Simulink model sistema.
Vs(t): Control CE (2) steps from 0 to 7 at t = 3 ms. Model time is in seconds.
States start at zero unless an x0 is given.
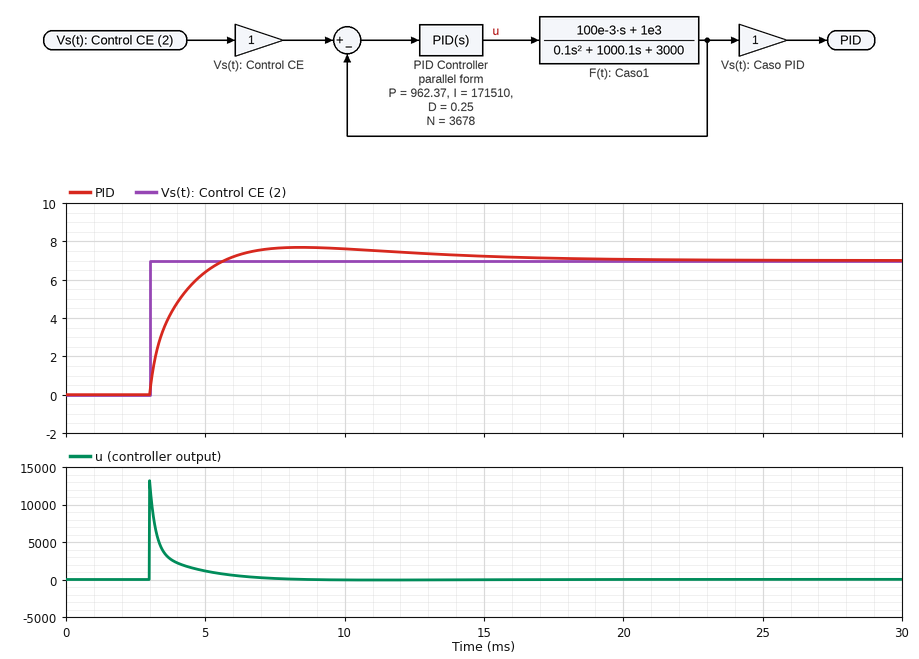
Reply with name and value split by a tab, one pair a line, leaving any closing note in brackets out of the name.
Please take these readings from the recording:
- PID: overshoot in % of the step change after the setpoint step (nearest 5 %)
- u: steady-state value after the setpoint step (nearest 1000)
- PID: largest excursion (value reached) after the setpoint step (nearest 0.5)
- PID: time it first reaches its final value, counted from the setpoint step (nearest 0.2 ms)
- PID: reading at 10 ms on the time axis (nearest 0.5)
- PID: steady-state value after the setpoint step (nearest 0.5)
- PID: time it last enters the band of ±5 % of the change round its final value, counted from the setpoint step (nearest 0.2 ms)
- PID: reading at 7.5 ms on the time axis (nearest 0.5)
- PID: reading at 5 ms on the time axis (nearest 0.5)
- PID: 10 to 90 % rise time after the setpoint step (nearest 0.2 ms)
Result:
PID: overshoot in % of the step change after the setpoint step	10 %
u: steady-state value after the setpoint step	0
PID: largest excursion (value reached) after the setpoint step	7.5
PID: time it first reaches its final value, counted from the setpoint step	2.6 ms
PID: reading at 10 ms on the time axis	7.5
PID: steady-state value after the setpoint step	7.0
PID: time it last enters the band of ±5 % of the change round its final value, counted from the setpoint step	10.0 ms
PID: reading at 7.5 ms on the time axis	7.5
PID: reading at 5 ms on the time axis	6.5
PID: 10 to 90 % rise time after the setpoint step	1.8 ms
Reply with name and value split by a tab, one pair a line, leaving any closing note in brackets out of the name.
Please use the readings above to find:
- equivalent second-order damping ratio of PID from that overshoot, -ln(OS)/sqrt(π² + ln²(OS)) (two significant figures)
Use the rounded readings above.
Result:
equivalent second-order damping ratio of PID from that overshoot, -ln(OS)/sqrt(π² + ln²(OS))	0.59
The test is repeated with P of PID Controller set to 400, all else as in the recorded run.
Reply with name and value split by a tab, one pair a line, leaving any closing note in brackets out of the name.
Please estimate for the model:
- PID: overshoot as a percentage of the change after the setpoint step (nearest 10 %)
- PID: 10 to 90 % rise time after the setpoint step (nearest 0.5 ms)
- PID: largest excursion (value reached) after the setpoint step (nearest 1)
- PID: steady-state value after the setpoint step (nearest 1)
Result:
PID: overshoot as a percentage of the change after the setpoint step	30 %
PID: 10 to 90 % rise time after the setpoint step	2.5 ms
PID: largest excursion (value reached) after the setpoint step	9
PID: steady-state value after the setpoint step	7
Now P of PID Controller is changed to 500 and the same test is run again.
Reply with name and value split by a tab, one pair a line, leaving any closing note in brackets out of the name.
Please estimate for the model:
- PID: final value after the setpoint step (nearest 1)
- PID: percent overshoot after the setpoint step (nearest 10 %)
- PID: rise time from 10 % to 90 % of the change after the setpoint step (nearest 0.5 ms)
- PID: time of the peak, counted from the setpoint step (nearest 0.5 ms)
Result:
PID: final value after the setpoint step	7
PID: percent overshoot after the setpoint step	20 %
PID: rise time from 10 % to 90 % of the change after the setpoint step	2.5 ms
PID: time of the peak, counted from the setpoint step	6.5 ms
